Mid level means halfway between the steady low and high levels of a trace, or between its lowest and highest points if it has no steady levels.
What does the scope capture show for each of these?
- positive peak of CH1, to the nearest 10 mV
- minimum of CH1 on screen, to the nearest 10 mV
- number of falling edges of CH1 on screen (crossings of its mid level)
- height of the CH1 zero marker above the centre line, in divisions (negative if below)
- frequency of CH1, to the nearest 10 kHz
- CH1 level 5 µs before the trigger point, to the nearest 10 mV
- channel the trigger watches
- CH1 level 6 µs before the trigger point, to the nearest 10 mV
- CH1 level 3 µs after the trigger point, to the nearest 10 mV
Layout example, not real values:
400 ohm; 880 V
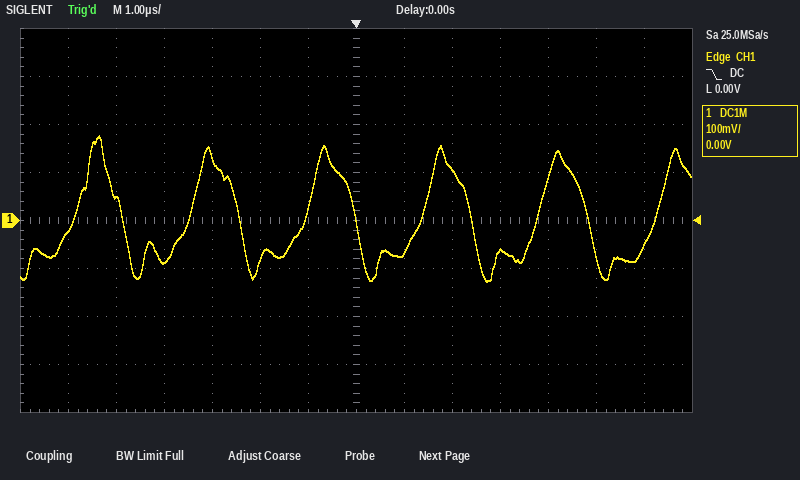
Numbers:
180 mV; -130 mV; 5; 0.0 div; 410 kHz; 50 mV; CH1; -20 mV; -60 mV
